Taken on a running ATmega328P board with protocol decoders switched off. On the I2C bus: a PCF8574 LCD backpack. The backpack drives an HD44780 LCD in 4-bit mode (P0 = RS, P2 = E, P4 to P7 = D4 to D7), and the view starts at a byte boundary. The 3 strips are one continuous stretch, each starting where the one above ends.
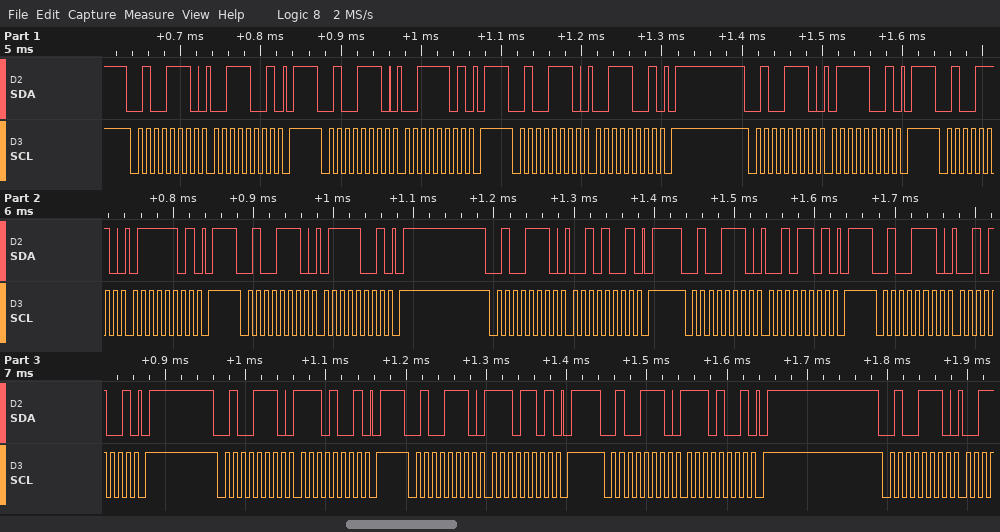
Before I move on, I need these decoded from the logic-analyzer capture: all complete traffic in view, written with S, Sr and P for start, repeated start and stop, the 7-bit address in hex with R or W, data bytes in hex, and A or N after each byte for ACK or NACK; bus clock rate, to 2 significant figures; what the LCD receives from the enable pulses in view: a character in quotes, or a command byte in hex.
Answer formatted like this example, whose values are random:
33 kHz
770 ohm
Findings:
S 27W A 39 A P S 27W A 3D A P S 27W A 39 A P S 27W A 79 A P S 27W A 7D A P S 27W A 79 A P S 27W A 29 A P S 27W A 2D A P S 27W A 29 A P S 27W A E9 A P S 27W A ED A P S 27W A E9 A P S 27W A
100 kHz
'7' '.'
